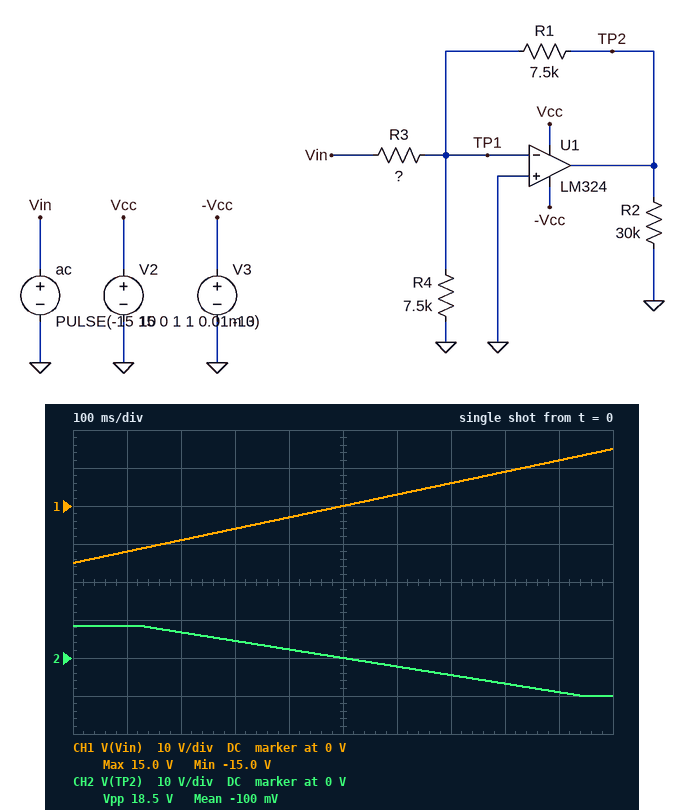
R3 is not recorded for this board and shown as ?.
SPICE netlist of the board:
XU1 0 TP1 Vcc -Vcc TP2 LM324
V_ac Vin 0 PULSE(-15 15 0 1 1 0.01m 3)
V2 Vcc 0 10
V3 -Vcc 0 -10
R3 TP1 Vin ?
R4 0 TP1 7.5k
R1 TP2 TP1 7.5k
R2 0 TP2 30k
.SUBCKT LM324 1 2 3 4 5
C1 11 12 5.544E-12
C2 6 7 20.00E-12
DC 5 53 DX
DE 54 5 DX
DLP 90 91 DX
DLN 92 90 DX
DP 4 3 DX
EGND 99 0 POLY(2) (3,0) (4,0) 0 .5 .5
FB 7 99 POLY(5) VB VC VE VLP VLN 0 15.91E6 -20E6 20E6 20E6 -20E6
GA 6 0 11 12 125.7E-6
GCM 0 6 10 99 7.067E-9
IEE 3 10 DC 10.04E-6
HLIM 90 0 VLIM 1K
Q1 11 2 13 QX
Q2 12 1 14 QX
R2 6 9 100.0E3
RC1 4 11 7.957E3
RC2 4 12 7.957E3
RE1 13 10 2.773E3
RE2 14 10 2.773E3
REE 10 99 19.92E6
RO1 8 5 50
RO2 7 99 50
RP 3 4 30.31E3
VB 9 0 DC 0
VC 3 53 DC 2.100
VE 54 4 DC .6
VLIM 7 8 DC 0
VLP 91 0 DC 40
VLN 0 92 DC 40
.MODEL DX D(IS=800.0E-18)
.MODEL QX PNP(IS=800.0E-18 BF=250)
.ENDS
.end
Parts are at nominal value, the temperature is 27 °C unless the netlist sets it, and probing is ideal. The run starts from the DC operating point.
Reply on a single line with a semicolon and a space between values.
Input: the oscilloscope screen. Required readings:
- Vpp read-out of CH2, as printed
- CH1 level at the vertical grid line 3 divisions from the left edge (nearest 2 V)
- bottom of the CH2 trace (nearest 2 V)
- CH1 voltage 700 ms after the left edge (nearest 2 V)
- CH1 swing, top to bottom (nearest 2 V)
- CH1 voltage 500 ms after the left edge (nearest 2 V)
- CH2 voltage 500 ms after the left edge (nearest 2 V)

18.5 V; -6 V; -10 V; 6 V; 30 V; 0 V; 0 V
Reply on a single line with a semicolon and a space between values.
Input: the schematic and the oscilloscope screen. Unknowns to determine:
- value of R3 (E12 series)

10 kΩ
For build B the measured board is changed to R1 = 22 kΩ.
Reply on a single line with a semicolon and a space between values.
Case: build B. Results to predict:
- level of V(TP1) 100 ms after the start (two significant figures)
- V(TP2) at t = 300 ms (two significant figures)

-2.9 V; 8.5 V
